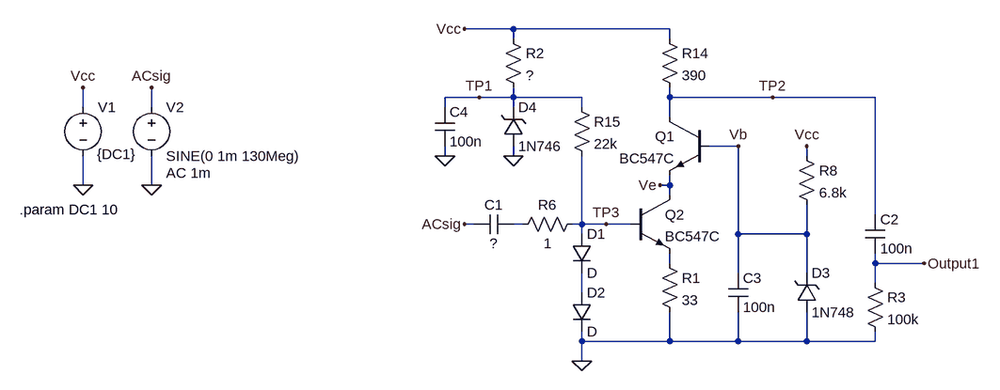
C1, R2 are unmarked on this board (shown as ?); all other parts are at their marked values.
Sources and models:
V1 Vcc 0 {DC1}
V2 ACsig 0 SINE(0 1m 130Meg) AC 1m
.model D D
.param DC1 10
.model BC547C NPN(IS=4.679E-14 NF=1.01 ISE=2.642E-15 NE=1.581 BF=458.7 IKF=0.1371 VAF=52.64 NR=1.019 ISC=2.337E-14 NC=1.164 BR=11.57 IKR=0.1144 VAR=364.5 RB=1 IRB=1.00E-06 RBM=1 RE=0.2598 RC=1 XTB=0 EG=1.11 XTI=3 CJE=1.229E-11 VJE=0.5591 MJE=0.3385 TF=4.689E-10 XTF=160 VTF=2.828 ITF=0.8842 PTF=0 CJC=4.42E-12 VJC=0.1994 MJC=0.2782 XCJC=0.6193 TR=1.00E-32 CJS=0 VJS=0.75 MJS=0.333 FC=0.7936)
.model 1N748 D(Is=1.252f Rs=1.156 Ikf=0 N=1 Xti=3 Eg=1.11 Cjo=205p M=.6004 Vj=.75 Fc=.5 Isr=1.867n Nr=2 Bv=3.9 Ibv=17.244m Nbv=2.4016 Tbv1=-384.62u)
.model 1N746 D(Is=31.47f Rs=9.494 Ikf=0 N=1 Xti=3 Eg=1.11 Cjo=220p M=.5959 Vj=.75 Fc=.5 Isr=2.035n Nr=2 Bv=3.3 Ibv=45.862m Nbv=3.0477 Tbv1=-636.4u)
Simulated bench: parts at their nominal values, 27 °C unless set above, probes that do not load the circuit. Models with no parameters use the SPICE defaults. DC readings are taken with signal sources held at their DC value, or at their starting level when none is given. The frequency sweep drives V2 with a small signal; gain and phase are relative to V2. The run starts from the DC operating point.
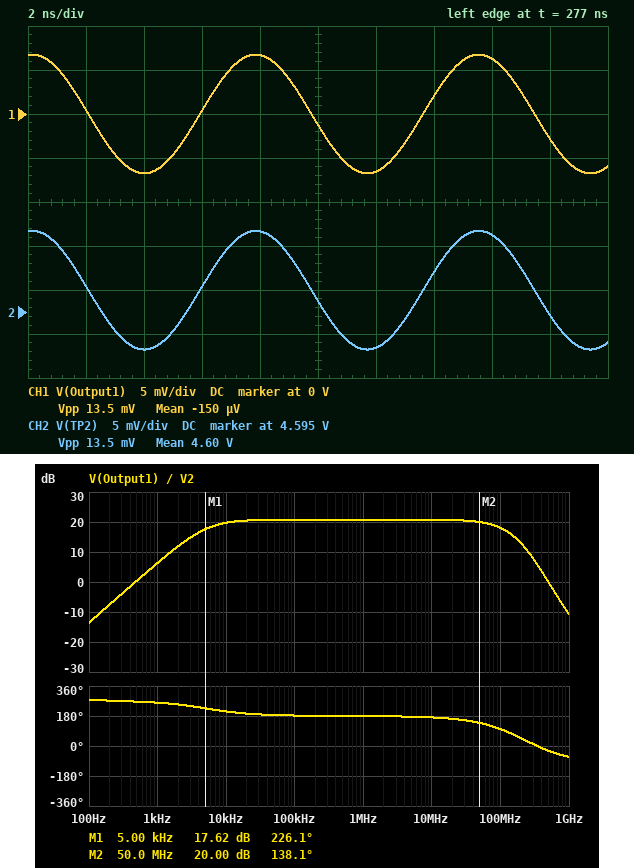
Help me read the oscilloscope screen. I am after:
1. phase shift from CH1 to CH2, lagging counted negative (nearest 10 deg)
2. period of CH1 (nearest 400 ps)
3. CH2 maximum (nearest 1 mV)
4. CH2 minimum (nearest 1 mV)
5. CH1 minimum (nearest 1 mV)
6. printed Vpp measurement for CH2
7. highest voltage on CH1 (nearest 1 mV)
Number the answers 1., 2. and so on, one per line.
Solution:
1. 0 deg
2. 7.6 ns
3. 4.604 V
4. 4.591 V
5. -7 mV
6. 13.5 mV
7. 7 mV
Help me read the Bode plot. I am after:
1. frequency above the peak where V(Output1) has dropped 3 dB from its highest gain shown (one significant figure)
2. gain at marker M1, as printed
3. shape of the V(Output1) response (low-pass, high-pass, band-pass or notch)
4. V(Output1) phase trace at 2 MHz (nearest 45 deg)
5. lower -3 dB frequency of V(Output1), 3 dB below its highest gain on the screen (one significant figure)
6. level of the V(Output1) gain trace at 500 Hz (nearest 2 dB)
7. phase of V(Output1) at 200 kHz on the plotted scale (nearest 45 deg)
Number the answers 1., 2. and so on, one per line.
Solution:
1. 100 MHz
2. 17.62 dB
3. band-pass
4. 180 deg
5. 5 kHz
6. 0 dB
7. 180 deg
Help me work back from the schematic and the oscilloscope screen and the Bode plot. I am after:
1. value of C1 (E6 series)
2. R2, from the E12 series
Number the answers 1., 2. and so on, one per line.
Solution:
1. 33 nF
2. 12 kΩ
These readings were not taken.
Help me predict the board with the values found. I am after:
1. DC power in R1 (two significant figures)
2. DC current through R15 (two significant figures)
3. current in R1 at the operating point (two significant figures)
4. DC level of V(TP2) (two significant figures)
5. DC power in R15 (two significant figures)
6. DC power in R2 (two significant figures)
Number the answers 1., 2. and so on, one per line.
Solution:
1. 6.4 mW
2. 82 µA
3. 14 mA
4. 4.6 V
5. 150 µW
6. 4.1 mW
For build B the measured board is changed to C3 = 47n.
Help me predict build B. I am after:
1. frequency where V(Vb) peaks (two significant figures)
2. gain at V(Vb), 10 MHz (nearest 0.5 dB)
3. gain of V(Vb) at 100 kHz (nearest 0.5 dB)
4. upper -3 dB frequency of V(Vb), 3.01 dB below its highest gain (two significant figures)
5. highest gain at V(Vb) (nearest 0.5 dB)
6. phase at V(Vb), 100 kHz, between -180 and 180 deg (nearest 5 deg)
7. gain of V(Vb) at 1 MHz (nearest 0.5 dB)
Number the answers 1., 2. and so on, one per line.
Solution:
1. 16 kHz
2. -60.0 dB
3. -51.5 dB
4. 60 kHz
5. -46.0 dB
6. 140 deg
7. -59.5 dB
